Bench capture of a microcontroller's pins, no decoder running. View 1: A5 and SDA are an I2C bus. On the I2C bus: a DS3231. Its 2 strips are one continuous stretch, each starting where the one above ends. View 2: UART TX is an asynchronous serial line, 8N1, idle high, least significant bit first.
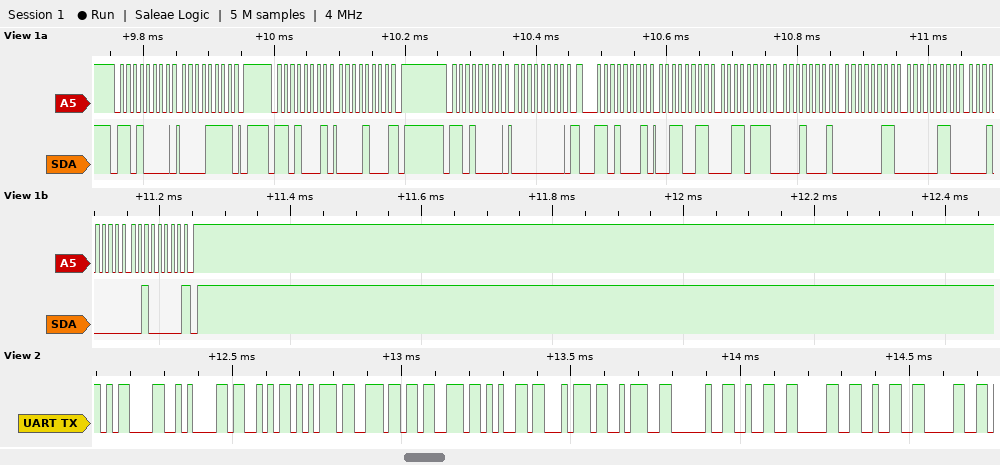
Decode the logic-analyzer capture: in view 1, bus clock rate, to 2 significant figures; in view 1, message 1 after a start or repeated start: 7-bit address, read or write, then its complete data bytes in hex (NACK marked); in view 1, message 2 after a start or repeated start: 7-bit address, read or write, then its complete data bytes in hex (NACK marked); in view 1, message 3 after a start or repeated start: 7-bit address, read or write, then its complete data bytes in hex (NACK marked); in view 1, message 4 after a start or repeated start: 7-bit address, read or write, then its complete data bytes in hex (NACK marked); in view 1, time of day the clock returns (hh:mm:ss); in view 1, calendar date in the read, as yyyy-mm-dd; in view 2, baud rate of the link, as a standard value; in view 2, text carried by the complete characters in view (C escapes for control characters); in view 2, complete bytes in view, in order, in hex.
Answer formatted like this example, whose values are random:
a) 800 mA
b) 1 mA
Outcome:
a) 100 kHz
b) 0x68 write: 0F
c) 0x68 read: 08 NACK
d) 0x68 write: 00
e) 0x68 read: 33 37 11 03 06 10 20 NACK
f) 11:37:33
g) 2020-10-06
h) 57600 baud
i) "\r\nSunset: 2020"
j) 0D 0A 53 75 6E 73 65 74 3A 20 32 30 32 30
